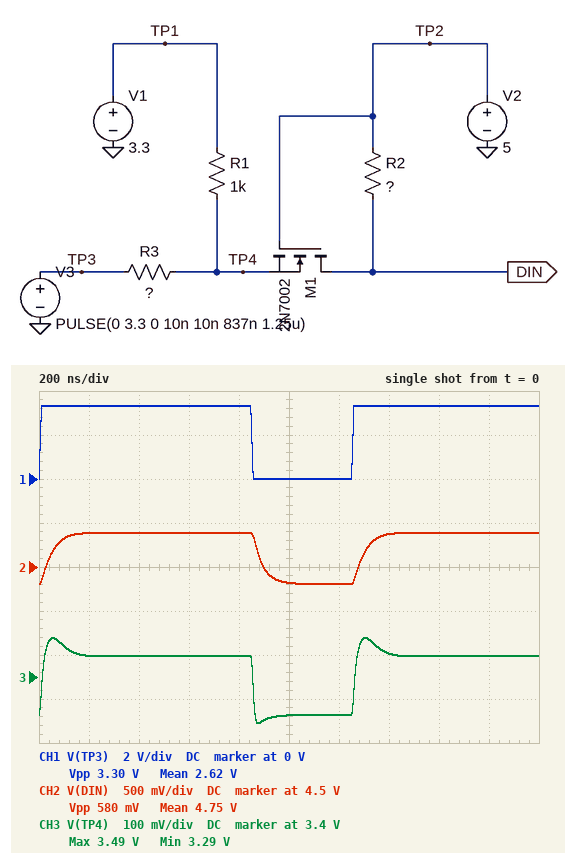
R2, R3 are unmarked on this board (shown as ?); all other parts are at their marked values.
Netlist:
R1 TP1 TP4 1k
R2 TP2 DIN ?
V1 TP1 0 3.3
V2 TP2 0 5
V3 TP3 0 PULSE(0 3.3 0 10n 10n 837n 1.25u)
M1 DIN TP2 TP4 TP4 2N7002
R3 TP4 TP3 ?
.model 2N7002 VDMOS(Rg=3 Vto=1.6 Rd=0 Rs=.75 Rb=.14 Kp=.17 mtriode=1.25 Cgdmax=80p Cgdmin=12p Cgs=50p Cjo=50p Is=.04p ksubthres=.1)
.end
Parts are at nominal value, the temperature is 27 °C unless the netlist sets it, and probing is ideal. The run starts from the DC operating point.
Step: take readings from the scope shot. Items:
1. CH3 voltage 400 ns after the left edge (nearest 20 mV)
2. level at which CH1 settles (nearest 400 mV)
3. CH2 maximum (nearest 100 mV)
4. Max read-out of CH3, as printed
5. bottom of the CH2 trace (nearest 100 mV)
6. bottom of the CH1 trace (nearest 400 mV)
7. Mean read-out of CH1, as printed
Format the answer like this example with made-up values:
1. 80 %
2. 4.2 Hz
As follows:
1. 3.44 V
2. 3.2 V
3. 4.9 V
4. 3.49 V
5. 4.3 V
6. 0 V
7. 2.62 V
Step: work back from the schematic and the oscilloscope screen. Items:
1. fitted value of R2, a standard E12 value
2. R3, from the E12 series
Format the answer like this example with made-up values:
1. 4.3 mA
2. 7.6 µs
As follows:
1. 560 Ω
2. 2.7 kΩ
